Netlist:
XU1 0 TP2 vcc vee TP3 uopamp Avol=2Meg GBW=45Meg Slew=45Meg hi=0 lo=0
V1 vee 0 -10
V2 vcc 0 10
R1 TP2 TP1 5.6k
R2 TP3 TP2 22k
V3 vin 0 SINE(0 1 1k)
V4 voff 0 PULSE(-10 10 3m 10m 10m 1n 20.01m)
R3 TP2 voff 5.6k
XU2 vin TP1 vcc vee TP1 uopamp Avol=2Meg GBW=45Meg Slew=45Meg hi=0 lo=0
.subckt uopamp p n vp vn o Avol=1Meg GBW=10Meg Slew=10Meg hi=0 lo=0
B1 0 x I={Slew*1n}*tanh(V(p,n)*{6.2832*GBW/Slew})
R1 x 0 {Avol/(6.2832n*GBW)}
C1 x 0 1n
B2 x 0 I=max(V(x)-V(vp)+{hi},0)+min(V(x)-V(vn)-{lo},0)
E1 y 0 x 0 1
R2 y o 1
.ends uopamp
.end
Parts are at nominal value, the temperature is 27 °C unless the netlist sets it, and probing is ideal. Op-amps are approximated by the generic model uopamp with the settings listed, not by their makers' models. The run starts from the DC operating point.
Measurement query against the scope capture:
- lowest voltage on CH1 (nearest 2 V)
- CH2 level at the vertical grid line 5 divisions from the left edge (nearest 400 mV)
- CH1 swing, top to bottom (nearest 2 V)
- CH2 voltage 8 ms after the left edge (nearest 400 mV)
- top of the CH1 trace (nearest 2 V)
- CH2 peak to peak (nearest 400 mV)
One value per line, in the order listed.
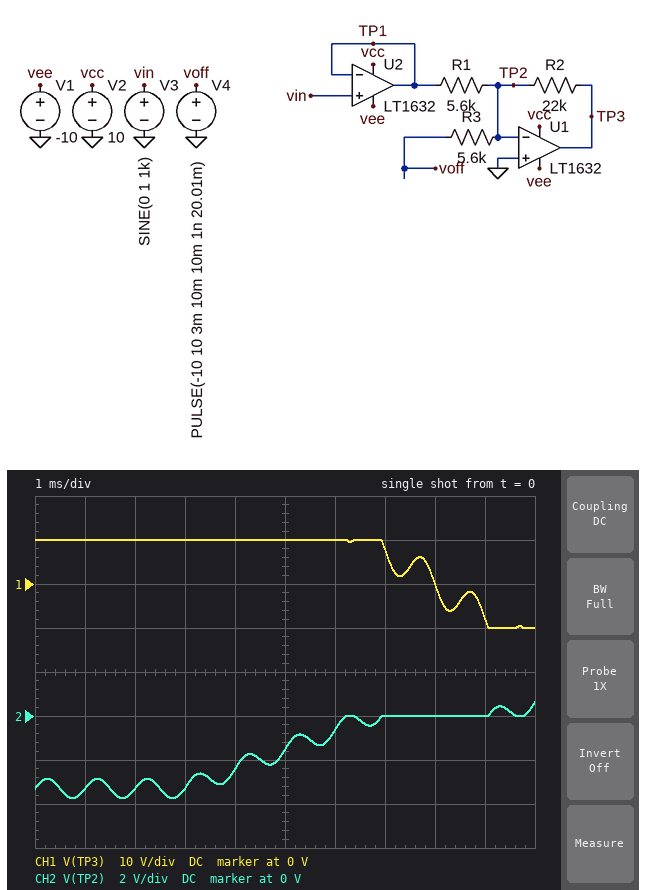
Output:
-10 V
-1.6 V
20 V
0 V
10 V
4.4 V
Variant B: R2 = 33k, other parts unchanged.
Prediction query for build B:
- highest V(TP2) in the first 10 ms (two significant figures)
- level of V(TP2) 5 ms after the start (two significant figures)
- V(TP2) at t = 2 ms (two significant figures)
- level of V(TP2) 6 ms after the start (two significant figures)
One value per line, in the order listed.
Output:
1.1 V
-2.0 V
-3.8 V
-1.1 V
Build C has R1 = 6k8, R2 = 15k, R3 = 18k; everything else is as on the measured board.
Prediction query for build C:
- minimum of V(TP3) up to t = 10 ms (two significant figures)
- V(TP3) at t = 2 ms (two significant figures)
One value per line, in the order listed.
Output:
-4.3 V
8.3 V
